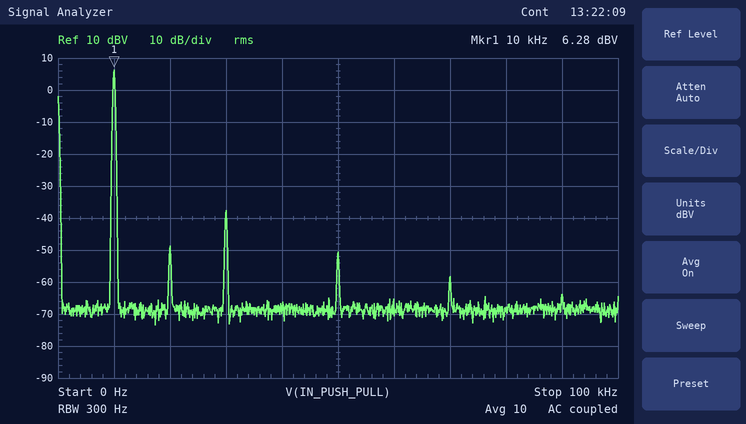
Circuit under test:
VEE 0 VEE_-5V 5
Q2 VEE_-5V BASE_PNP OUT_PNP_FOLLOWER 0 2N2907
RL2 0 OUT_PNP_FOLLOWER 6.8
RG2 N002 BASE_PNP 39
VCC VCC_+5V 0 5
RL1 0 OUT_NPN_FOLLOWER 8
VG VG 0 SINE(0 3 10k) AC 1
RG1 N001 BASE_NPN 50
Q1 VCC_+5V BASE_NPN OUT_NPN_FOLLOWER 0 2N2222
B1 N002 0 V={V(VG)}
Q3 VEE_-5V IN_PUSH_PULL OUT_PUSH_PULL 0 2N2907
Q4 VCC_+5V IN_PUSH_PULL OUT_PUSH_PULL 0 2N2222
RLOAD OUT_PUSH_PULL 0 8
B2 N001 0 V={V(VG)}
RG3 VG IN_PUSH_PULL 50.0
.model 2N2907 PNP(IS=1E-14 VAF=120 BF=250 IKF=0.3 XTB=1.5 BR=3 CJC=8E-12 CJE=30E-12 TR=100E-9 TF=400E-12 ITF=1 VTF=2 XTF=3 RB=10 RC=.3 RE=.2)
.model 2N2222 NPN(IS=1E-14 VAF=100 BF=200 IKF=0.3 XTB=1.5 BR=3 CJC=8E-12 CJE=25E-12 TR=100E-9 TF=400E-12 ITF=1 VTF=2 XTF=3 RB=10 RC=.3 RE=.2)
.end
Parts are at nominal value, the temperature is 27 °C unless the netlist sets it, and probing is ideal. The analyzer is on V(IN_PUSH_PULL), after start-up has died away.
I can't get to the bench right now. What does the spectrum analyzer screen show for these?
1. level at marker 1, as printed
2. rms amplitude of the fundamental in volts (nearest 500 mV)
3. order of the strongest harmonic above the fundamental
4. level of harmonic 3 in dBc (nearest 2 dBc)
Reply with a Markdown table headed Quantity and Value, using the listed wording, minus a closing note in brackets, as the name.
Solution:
| Quantity | Value |
|---|---|
| level at marker 1, as printed | 6.28 dBV |
| rms amplitude of the fundamental in volts | 2.0 V |
| order of the strongest harmonic above the fundamental | 3 |
| level of harmonic 3 in dBc | -44 dBc |
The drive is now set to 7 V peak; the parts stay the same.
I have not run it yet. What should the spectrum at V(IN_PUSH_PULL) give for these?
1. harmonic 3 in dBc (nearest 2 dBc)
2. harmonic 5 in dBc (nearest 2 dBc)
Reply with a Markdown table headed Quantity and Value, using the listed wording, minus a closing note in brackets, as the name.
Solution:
| Quantity | Value |
|---|---|
| harmonic 3 in dBc | -26 dBc |
| harmonic 5 in dBc | -34 dBc |
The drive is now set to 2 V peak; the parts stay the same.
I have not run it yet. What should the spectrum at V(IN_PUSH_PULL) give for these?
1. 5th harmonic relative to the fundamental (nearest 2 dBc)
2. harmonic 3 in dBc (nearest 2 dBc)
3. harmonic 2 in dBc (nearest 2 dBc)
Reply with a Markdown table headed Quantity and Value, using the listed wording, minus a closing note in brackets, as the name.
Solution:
| Quantity | Value |
|---|---|
| 5th harmonic relative to the fundamental | -60 dBc |
| harmonic 3 in dBc | -46 dBc |
| harmonic 2 in dBc | -58 dBc |
